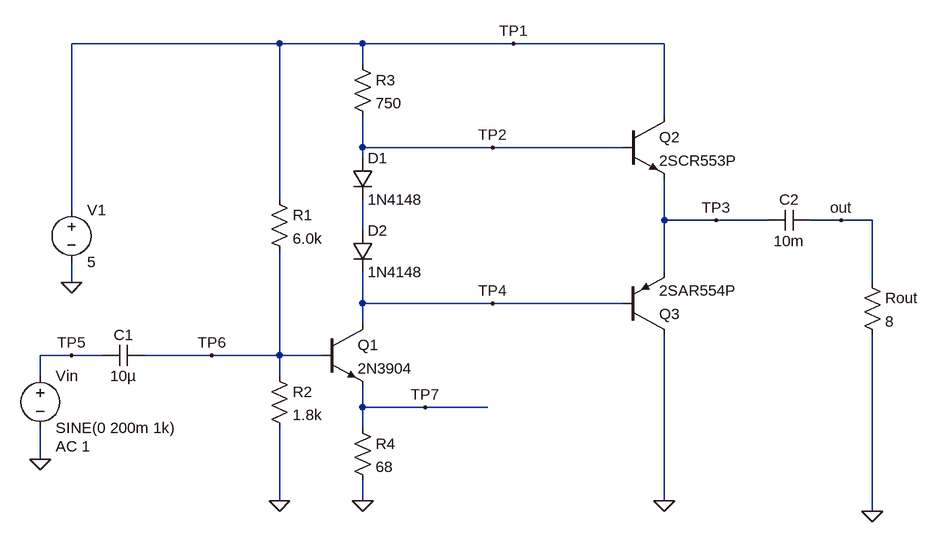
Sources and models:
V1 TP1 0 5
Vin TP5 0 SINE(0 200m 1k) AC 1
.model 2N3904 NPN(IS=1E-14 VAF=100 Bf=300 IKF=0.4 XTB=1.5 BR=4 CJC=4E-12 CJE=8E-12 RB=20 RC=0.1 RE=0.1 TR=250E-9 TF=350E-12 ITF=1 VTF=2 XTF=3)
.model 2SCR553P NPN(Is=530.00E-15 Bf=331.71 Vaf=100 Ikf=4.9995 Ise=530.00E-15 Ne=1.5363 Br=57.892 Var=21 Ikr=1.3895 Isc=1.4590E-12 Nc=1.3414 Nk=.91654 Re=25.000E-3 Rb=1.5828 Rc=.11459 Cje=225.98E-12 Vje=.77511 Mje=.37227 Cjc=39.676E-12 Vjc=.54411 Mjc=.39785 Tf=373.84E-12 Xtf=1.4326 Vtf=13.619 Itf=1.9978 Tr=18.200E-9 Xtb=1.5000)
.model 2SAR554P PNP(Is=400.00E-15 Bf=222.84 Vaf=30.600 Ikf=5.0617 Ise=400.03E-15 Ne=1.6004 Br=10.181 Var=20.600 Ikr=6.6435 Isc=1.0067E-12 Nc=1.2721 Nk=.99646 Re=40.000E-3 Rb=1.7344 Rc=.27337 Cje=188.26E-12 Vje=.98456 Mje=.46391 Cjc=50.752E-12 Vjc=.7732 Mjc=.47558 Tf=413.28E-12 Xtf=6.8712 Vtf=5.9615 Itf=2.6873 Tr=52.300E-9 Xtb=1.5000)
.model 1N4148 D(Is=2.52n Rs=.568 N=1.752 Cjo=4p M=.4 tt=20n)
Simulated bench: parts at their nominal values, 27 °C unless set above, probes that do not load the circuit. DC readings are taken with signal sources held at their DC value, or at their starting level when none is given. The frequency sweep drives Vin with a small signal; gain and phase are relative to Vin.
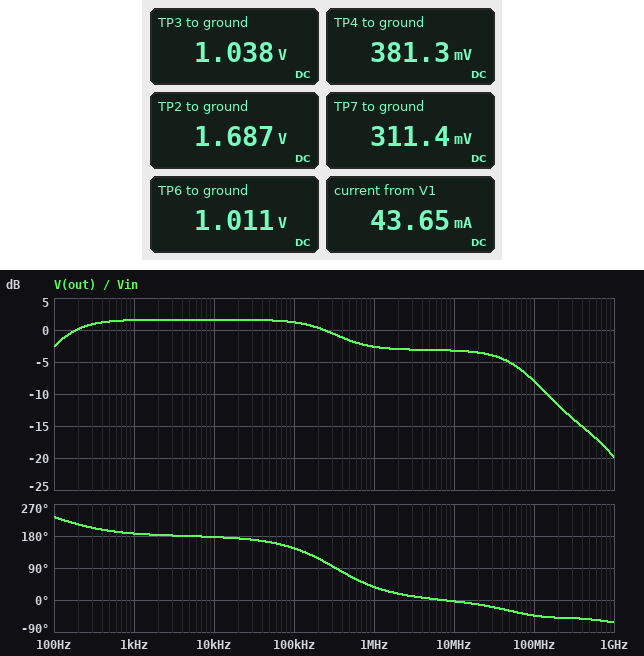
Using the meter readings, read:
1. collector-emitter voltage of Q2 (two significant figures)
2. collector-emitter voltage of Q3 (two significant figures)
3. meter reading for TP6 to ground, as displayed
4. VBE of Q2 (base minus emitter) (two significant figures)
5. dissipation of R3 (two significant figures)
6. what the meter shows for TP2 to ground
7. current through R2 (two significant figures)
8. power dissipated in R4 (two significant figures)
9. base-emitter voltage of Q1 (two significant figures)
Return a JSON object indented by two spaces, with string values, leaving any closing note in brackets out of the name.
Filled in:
{
  "collector-emitter voltage of Q2": "4.0 V",
  "collector-emitter voltage of Q3": "-1.0 V",
  "meter reading for TP6 to ground, as displayed": "1.011 V",
  "VBE of Q2 (base minus emitter)": "650 mV",
  "dissipation of R3": "15 mW",
  "what the meter shows for TP2 to ground": "1.687 V",
  "current through R2": "560 µA",
  "power dissipated in R4": "1.4 mW",
  "base-emitter voltage of Q1": "700 mV"
}
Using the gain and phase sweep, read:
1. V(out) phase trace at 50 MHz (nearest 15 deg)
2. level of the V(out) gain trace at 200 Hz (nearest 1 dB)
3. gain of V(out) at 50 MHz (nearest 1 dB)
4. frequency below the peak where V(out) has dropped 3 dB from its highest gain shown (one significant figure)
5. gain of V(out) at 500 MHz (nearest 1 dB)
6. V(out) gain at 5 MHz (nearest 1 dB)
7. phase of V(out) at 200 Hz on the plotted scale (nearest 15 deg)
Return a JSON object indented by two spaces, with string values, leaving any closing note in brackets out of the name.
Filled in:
{
  "V(out) phase trace at 50 MHz": "-30 deg",
  "level of the V(out) gain trace at 200 Hz": "0 dB",
  "gain of V(out) at 50 MHz": "-5 dB",
  "frequency below the peak where V(out) has dropped 3 dB from its highest gain shown": "100 Hz",
  "gain of V(out) at 500 MHz": "-16 dB",
  "V(out) gain at 5 MHz": "-3 dB",
  "phase of V(out) at 200 Hz on the plotted scale": "210 deg"
}
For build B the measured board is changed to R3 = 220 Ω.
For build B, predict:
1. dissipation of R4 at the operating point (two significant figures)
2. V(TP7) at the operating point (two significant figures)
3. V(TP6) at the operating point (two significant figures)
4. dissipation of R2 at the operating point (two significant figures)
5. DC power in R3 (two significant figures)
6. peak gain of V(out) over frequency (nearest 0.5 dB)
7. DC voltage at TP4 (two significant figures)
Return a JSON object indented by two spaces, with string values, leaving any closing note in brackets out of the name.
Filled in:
{
  "dissipation of R4 at the operating point": "2.6 mW",
  "V(TP7) at the operating point": "420 mV",
  "V(TP6) at the operating point": "1.1 V",
  "dissipation of R2 at the operating point": "700 µW",
  "DC power in R3": "8.2 mW",
  "peak gain of V(out) over frequency": "8.5 dB",
  "DC voltage at TP4": "2.3 V"
}
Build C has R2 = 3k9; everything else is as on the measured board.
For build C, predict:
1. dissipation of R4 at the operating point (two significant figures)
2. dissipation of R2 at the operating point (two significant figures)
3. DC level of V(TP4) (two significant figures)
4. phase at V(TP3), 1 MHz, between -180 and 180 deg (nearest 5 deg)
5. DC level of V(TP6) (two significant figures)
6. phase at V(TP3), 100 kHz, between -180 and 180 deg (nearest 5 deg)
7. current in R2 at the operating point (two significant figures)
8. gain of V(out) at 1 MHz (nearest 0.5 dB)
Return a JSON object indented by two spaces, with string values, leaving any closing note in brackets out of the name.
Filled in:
{
  "dissipation of R4 at the operating point": "1.6 mW",
  "dissipation of R2 at the operating point": "280 µW",
  "DC level of V(TP4)": "370 mV",
  "phase at V(TP3), 1 MHz, between -180 and 180 deg": "10 deg",
  "DC level of V(TP6)": "1.0 V",
  "phase at V(TP3), 100 kHz, between -180 and 180 deg": "40 deg",
  "current in R2 at the operating point": "270 µA",
  "gain of V(out) at 1 MHz": "-3.0 dB"
}
